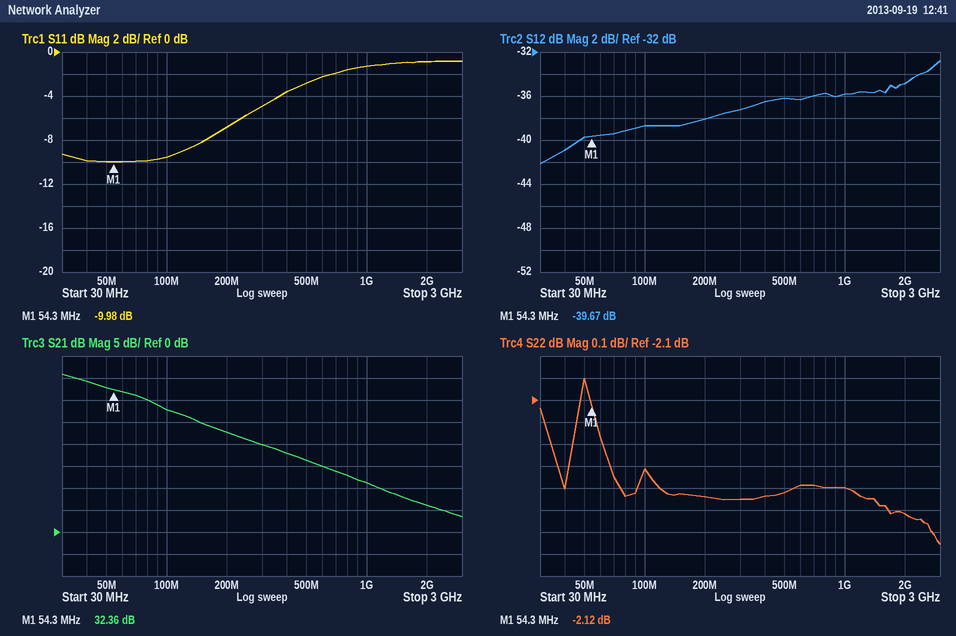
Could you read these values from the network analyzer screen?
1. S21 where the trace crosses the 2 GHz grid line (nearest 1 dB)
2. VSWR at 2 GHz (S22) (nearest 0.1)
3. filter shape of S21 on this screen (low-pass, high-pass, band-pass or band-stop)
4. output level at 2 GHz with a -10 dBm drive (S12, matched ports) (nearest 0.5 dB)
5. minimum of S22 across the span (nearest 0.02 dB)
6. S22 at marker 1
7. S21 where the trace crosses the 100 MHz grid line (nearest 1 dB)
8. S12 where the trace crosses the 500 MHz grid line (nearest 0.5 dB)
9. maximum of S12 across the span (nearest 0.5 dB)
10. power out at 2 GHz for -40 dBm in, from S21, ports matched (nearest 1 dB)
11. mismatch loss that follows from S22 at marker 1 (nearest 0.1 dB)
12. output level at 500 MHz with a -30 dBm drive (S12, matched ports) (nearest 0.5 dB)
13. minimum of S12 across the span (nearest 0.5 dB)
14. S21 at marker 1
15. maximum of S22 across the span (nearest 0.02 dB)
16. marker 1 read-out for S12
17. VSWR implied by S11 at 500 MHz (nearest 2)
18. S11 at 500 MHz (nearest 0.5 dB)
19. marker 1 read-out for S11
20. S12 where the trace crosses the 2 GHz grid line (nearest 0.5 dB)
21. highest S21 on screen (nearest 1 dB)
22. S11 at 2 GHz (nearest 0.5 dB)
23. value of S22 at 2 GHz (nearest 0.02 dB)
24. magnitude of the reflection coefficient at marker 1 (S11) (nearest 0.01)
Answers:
6 dB
6.7
low-pass
-45.0 dBm
-2.76 dB
-2.12 dB
28 dB
-36.0 dB
-33.0 dB
-34 dBm
4.1 dB
-66.0 dBm
-42.0 dB
32.36 dB
-2.00 dB
-39.67 dB
6
-3.0 dB
-9.98 dB
-35.0 dB
36 dB
-1.0 dB
-2.62 dB
0.32
